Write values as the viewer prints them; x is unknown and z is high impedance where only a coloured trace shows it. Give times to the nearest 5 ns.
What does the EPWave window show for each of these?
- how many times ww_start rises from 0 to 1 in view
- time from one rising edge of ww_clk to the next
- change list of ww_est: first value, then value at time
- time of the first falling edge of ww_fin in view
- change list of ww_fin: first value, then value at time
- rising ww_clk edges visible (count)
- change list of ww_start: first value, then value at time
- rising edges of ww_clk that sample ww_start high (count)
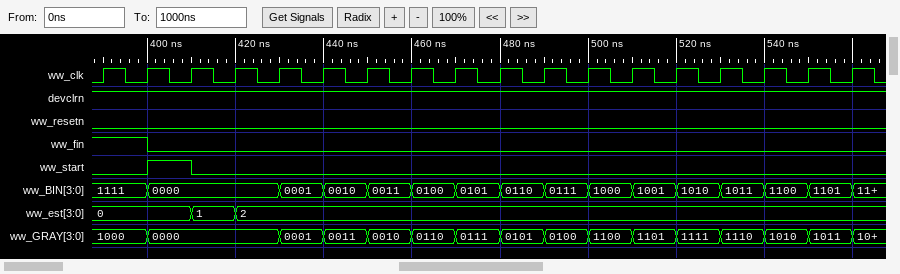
1
10 ns
0, 1 at 410 ns, 2 at 420 ns
400 ns
1, 0 at 400 ns
18
0, 1 at 400 ns, 0 at 410 ns
1
